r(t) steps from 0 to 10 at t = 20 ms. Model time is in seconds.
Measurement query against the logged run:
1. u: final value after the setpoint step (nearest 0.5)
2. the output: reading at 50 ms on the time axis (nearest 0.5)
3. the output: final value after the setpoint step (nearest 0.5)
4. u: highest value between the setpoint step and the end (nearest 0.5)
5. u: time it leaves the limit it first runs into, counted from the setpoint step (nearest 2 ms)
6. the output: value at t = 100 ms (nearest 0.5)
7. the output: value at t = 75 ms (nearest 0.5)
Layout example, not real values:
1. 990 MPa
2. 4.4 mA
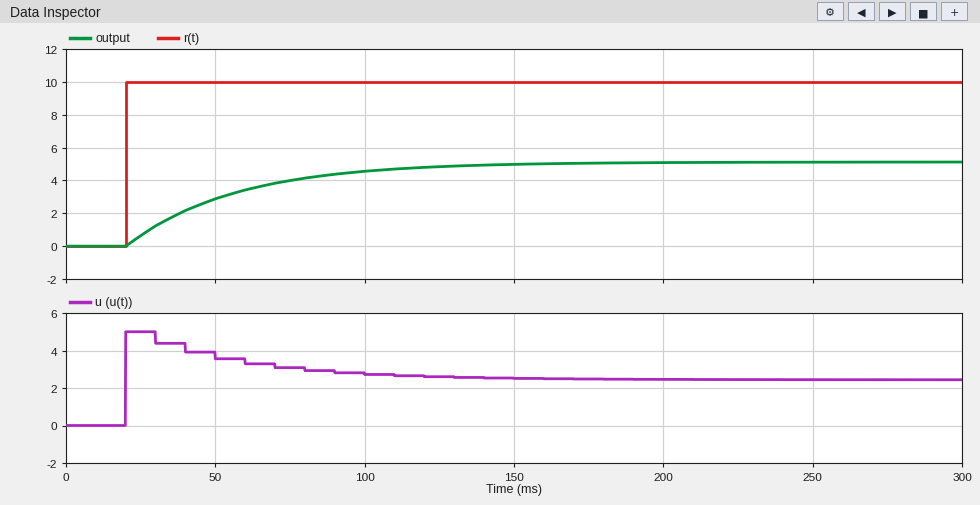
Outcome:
1. 2.5
2. 3.0
3. 5.0
4. 5.0
5. 10 ms
6. 4.5
7. 4.0
